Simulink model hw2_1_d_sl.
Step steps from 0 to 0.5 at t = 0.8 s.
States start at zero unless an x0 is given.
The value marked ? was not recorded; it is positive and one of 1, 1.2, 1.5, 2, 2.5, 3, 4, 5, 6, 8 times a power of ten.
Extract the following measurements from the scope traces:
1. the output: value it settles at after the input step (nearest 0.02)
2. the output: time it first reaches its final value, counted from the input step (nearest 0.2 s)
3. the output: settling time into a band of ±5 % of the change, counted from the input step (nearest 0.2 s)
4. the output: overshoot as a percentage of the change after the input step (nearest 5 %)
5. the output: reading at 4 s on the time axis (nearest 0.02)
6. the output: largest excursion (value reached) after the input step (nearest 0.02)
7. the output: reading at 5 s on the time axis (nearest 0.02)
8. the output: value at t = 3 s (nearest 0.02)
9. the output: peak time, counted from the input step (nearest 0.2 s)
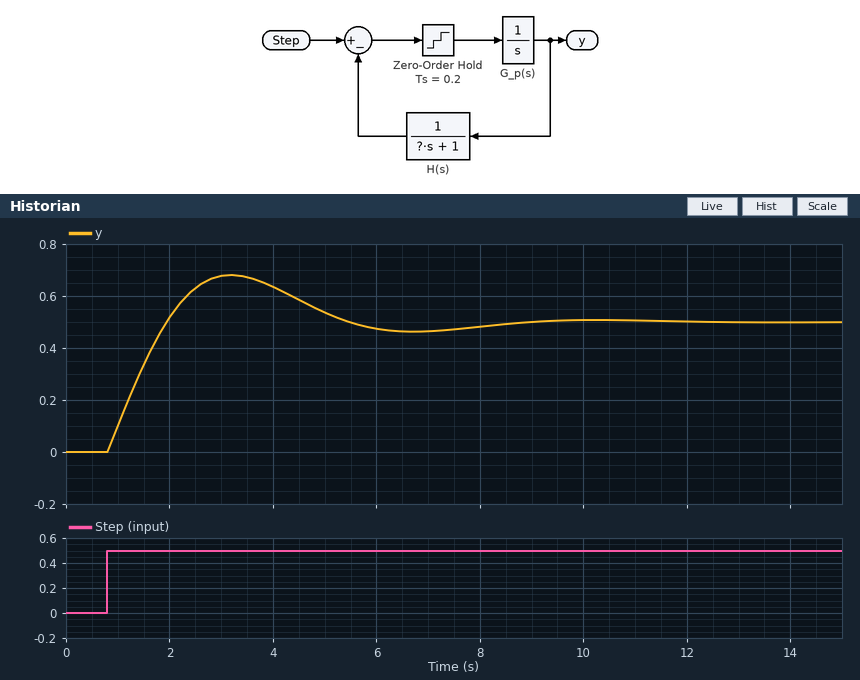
0.50
1.2 s
6.8 s
35 %
0.64
0.68
0.54
0.68
2.4 s
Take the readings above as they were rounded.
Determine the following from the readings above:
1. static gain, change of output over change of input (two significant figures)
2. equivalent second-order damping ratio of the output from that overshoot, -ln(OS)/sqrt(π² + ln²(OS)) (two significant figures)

1.0
0.32
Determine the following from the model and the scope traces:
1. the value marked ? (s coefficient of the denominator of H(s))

1
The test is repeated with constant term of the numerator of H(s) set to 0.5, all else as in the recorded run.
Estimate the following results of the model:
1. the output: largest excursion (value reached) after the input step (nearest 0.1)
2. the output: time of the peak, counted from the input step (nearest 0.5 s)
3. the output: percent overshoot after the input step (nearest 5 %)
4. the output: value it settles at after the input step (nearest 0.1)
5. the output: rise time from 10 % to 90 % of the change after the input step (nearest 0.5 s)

1.1
4.5 s
10 %
1.0
2.0 s
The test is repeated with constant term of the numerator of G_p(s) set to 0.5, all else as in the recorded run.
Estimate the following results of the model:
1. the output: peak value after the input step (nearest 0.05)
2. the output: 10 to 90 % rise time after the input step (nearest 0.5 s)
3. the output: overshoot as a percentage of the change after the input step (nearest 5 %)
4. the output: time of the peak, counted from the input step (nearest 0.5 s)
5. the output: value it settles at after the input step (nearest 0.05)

0.55
2.0 s
10 %
4.5 s
0.50
